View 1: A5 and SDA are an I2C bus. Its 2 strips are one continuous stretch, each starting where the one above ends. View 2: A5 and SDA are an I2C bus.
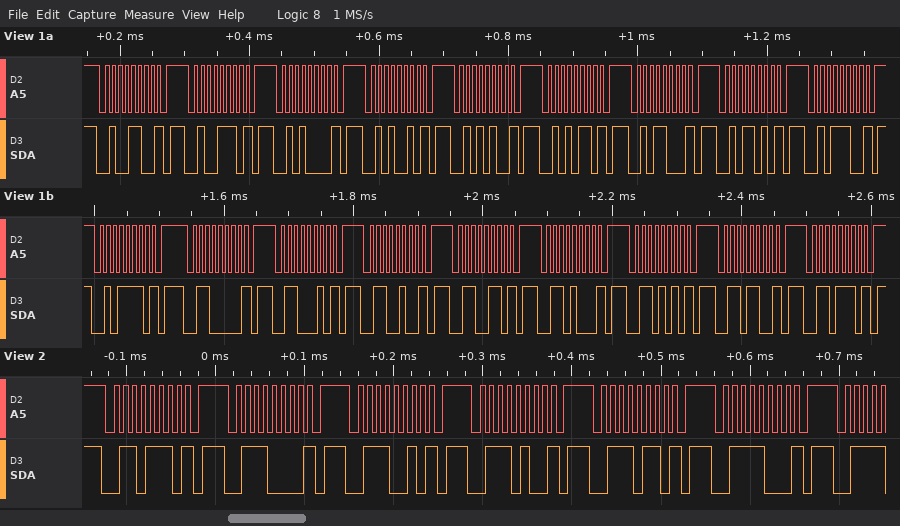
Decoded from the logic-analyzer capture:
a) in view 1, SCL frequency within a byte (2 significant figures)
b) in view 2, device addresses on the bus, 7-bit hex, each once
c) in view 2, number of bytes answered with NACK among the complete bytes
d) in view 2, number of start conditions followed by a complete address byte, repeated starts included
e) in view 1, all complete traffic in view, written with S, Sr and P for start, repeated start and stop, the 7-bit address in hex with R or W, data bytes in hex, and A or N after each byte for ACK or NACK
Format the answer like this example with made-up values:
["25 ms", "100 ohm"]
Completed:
["100 kHz", "0x37 0x38 0x39 0x3A 0x3B 0x3C", "6", "6", "S 26W N P S 27W N P S 28W N P S 29W N P S 2AW N P S 2BW N P S 2CW N P S 2DW N P S 2EW N P S 2FW N P S 30W N P S 31W N P S 32W N P S 33W N P S 34W N P S 35W N P S 36W N P S 37W N P"]
